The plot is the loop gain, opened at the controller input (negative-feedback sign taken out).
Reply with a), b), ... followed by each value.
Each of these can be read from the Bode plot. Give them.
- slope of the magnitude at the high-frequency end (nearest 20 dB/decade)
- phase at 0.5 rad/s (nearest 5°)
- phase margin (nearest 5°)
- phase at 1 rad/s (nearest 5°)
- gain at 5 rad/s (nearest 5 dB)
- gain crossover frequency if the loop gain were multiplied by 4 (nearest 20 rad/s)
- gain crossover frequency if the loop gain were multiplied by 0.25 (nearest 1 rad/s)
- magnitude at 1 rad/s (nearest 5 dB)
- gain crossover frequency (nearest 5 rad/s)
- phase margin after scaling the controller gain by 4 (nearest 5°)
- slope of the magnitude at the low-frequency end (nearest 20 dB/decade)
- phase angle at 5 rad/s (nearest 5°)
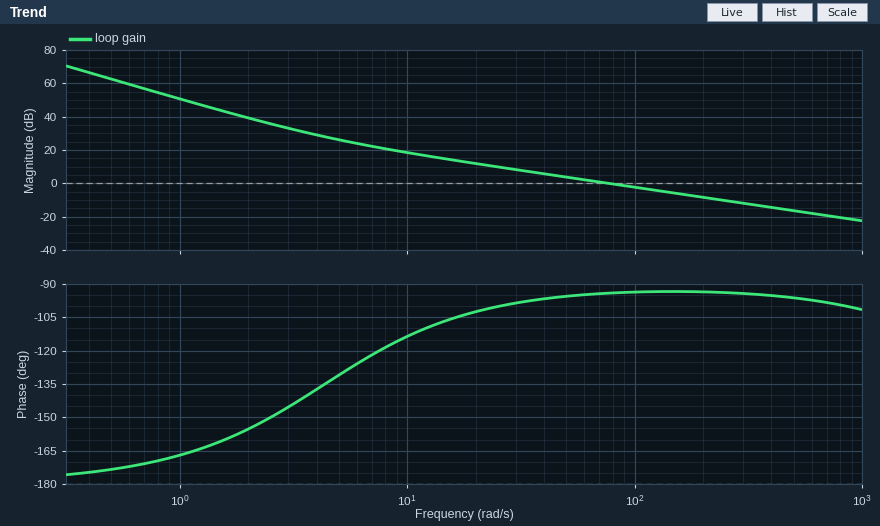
a) -20 dB/decade
b) -175°
c) 85°
d) -165°
e) 25 dB
f) 300 rad/s
g) 20 rad/s
h) 50 dB
i) 75 rad/s
j) 85°
k) -40 dB/decade
l) -130°
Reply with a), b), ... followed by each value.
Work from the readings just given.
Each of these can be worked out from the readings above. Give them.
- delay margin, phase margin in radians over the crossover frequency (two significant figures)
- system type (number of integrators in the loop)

a) 0.020 s
b) 2
